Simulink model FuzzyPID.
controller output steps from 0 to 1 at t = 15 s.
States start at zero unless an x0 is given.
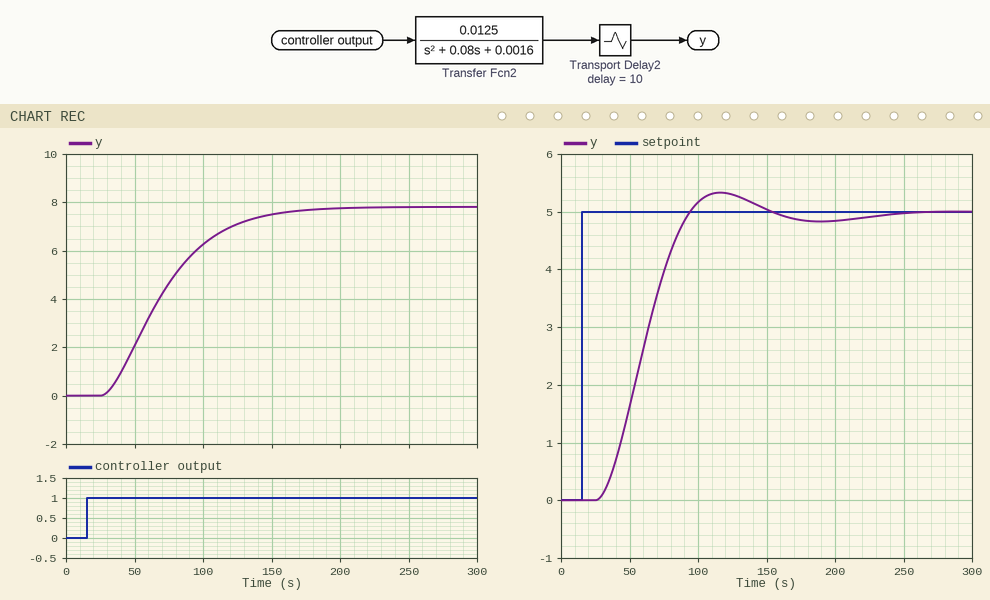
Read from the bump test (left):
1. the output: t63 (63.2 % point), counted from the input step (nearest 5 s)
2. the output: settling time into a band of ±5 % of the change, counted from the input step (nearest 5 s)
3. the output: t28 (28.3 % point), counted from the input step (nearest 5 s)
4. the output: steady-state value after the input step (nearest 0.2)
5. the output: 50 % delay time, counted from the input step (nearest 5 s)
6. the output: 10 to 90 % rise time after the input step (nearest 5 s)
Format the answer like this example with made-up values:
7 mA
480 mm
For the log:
65 s
130 s
35 s
7.8
50 s
85 s
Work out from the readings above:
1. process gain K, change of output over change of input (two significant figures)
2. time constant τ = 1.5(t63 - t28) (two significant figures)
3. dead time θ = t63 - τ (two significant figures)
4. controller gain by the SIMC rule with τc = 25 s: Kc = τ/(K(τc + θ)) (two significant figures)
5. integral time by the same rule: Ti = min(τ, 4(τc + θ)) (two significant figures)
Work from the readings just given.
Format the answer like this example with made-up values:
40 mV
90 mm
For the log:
7.8
45 s
20 s
0.13
45 s
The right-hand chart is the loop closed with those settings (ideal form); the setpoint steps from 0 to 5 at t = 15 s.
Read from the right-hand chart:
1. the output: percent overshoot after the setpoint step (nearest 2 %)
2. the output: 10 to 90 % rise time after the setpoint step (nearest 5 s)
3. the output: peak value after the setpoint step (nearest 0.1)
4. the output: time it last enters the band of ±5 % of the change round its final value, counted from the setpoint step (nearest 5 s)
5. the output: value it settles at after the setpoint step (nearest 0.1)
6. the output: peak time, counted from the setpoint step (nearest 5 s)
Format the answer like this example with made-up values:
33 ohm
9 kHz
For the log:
6 %
45 s
5.3
115 s
5.0
100 s
